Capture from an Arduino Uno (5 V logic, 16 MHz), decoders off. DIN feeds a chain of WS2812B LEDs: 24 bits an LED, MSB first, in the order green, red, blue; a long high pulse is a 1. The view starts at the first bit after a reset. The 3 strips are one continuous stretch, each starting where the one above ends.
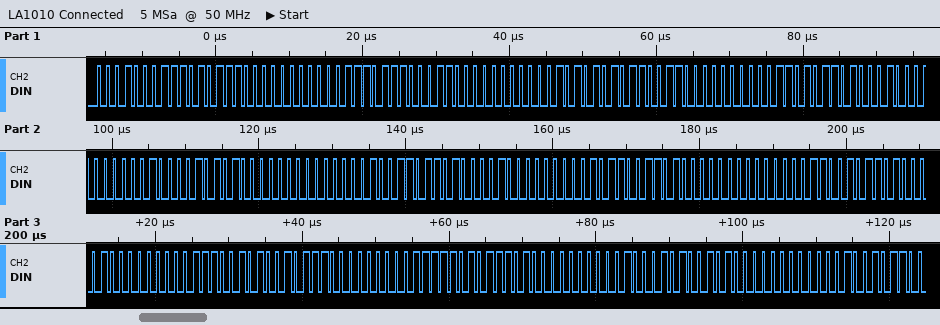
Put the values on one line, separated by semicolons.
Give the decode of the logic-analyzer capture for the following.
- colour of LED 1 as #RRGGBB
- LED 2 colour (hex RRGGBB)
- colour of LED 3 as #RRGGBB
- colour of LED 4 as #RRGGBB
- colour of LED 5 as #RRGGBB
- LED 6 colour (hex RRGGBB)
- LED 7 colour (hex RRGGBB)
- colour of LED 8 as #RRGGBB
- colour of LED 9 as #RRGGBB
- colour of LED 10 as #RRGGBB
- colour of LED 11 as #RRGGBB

#D71100; #C61D00; #B32A00; #A23500; #A04200; #A14D00; #A05900; #A16500; #977200; #747D00; #508A00
